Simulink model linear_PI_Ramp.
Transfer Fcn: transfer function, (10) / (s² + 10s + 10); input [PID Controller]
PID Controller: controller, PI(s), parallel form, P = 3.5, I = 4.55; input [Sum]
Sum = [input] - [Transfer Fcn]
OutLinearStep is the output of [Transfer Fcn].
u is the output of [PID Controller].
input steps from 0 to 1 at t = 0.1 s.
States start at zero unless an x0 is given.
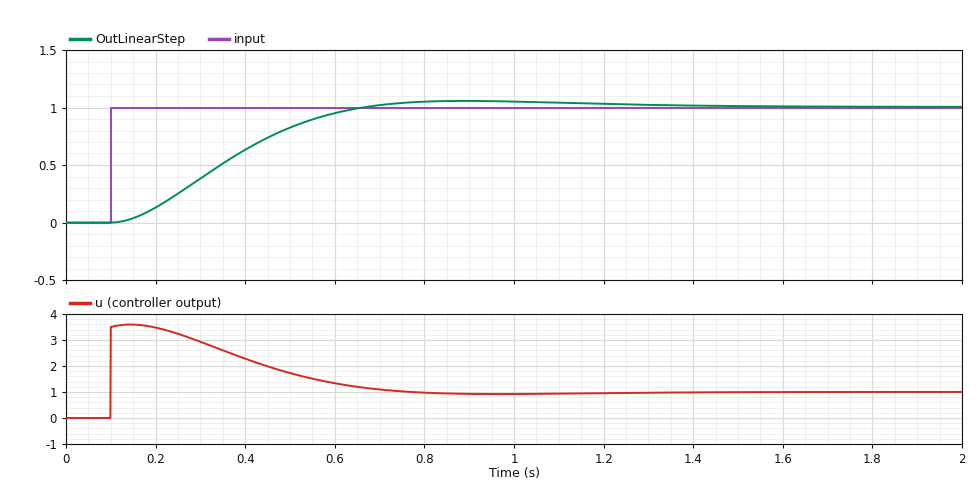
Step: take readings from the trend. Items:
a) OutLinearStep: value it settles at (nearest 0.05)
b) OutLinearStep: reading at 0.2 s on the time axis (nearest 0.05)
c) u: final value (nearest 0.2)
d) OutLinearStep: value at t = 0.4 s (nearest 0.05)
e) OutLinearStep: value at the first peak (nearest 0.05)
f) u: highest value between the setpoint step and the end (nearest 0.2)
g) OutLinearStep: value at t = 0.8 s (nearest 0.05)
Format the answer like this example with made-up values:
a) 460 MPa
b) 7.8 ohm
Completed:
a) 1.00
b) 0.15
c) 1.0
d) 0.65
e) 1.05
f) 3.6
g) 1.05
